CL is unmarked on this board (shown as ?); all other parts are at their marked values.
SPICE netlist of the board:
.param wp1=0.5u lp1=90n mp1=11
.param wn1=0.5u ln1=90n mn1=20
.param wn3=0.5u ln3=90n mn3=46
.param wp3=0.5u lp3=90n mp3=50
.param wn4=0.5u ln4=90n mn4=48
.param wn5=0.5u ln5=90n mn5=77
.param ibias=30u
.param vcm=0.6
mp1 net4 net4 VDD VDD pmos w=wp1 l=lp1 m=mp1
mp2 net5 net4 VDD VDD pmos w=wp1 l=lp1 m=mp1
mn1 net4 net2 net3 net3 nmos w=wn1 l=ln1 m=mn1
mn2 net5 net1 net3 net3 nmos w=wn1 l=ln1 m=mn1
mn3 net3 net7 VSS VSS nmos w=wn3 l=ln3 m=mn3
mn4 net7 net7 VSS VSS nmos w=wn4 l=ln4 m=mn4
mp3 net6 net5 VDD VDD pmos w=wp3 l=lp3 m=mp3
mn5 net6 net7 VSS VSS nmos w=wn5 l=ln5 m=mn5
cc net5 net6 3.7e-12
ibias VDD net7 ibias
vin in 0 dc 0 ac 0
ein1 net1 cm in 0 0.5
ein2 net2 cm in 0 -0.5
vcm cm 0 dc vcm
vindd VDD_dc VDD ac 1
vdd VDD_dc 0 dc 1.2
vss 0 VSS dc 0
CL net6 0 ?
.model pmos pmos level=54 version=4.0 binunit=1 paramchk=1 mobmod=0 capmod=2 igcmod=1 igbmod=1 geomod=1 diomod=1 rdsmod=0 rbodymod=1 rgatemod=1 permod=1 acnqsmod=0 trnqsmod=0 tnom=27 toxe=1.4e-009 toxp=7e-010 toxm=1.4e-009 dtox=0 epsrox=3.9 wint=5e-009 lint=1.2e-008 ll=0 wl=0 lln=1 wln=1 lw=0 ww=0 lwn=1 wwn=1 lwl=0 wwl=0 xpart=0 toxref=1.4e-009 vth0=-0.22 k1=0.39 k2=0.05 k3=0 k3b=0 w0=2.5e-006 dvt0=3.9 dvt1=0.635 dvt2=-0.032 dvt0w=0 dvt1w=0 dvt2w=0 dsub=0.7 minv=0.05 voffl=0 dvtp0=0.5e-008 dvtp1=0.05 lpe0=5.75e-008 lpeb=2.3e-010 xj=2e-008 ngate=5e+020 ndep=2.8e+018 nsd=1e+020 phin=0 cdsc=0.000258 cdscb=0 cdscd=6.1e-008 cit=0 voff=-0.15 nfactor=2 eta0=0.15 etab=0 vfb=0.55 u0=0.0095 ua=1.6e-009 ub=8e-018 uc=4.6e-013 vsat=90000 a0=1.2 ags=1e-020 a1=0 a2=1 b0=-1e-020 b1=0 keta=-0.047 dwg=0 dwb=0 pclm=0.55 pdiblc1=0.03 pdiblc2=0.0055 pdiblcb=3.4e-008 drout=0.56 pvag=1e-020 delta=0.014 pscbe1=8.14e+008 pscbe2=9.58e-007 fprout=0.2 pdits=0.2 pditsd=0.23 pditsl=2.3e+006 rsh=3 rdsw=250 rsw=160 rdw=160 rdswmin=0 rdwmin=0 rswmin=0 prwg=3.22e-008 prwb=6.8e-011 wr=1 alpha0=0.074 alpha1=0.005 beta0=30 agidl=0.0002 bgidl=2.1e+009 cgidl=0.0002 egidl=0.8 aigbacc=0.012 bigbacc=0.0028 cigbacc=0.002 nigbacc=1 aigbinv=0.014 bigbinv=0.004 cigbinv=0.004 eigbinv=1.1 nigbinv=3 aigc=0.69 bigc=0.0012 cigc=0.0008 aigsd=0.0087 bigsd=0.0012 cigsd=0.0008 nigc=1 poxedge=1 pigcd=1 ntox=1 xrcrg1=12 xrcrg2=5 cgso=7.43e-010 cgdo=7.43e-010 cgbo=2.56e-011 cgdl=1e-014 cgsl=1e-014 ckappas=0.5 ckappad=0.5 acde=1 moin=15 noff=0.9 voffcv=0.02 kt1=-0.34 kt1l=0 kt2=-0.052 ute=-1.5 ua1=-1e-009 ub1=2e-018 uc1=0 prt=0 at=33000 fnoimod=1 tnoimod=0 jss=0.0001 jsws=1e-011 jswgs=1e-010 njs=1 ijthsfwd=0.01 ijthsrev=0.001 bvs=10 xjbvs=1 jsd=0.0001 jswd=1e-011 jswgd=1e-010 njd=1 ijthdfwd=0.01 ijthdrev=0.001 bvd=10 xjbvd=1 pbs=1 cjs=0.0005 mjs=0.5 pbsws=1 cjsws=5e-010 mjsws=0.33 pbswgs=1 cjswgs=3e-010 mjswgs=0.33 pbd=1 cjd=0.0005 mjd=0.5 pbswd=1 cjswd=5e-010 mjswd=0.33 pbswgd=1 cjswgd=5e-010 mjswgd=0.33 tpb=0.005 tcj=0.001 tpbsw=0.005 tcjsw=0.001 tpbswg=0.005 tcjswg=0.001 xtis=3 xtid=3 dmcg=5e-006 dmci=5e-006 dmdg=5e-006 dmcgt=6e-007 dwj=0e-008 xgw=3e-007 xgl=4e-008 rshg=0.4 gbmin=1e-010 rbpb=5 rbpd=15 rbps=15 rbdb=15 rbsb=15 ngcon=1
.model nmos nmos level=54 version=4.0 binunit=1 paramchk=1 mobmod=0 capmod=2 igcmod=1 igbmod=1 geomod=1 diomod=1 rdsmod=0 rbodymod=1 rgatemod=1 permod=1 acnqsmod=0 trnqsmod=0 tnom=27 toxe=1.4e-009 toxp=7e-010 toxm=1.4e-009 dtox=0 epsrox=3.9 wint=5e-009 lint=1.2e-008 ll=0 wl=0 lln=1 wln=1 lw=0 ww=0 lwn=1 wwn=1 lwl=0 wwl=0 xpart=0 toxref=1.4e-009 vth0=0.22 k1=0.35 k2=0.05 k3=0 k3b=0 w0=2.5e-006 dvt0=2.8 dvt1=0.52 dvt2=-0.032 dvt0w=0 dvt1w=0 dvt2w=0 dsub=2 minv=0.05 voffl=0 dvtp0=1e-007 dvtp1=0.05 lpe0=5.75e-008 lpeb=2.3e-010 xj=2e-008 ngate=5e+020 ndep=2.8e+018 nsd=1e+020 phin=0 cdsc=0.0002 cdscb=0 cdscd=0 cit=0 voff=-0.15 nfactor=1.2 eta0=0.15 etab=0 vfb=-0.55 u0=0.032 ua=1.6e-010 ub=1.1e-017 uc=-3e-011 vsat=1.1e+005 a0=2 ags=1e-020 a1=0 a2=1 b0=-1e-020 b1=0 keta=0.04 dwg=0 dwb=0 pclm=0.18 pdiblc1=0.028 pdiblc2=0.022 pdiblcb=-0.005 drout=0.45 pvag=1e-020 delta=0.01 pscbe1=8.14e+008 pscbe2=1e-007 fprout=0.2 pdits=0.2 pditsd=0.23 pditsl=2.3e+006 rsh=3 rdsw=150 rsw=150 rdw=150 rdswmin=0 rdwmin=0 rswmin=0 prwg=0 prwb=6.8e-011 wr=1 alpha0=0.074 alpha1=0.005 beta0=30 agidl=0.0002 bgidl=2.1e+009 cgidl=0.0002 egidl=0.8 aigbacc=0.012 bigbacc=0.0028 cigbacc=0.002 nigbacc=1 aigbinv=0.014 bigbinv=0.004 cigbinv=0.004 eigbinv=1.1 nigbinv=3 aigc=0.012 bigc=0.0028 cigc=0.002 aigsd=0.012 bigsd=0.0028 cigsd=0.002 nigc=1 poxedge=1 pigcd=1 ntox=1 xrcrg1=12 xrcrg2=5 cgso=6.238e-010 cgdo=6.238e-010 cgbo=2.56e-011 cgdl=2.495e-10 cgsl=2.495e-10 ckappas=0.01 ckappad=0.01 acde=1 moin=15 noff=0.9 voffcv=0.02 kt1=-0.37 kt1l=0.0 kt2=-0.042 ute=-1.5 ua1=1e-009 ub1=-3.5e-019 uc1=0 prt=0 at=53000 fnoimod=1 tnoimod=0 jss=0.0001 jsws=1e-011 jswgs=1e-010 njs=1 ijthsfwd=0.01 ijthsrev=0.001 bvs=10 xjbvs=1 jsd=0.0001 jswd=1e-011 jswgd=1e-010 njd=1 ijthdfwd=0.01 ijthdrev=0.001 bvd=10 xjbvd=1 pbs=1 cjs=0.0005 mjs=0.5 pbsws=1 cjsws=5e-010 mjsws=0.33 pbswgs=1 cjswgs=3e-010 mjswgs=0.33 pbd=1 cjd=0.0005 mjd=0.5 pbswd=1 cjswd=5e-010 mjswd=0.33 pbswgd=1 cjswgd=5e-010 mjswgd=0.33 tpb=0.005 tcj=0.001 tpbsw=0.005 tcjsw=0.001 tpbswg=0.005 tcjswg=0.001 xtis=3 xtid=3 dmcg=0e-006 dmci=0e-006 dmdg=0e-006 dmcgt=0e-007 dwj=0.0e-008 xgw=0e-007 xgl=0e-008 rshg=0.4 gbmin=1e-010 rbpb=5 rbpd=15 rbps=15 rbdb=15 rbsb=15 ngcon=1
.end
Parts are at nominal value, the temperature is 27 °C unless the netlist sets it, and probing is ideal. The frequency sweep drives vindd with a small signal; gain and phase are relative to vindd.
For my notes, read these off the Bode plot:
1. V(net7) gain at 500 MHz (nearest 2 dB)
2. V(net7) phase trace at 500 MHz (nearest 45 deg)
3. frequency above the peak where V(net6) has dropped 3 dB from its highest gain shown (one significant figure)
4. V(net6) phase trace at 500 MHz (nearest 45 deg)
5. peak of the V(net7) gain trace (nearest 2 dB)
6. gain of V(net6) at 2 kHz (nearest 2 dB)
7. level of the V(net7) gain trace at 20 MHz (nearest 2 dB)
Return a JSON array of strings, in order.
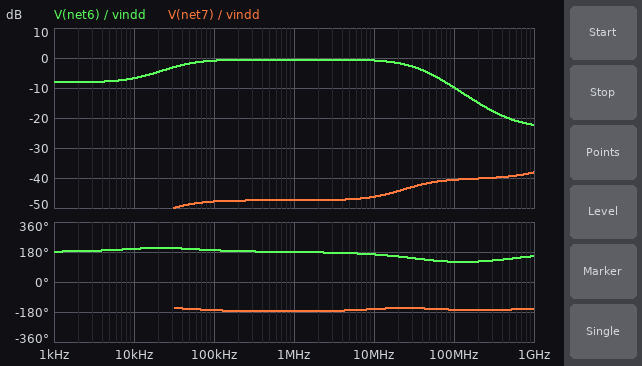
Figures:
["-40 dB", "-180 deg", "40 MHz", "135 deg", "-38 dB", "-8 dB", "-44 dB"]
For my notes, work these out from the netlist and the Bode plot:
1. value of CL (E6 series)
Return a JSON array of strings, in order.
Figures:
["4.7 pF"]
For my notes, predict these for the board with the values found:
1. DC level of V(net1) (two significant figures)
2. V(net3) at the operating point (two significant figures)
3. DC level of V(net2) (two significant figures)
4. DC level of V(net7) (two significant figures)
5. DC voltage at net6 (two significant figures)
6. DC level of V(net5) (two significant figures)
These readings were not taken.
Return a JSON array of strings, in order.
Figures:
["600 mV", "300 mV", "600 mV", "300 mV", "760 mV", "830 mV"]
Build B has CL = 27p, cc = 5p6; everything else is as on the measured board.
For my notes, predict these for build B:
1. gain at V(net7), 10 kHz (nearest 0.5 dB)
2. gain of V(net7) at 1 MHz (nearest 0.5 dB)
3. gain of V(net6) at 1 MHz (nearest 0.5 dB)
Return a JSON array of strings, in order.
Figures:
["-52.5 dB", "-48.0 dB", "-1.0 dB"]
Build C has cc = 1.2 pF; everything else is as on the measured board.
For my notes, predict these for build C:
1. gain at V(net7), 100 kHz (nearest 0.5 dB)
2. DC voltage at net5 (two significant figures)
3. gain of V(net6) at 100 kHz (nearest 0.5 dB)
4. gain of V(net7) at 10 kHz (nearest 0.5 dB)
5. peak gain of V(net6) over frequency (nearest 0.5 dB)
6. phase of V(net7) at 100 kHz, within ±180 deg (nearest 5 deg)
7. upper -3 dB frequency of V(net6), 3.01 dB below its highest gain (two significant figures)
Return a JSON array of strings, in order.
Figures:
["-50.0 dB", "830 mV", "-3.0 dB", "-55.0 dB", "-1.0 dB", "-160 deg", "35 MHz"]
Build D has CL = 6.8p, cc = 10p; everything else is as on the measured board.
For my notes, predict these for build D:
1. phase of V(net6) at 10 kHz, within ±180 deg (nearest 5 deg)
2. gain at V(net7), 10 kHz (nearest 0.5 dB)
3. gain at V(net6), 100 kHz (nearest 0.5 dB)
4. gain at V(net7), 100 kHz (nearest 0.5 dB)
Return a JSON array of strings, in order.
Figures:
["-155 deg", "-50.5 dB", "-0.5 dB", "-47.5 dB"]
